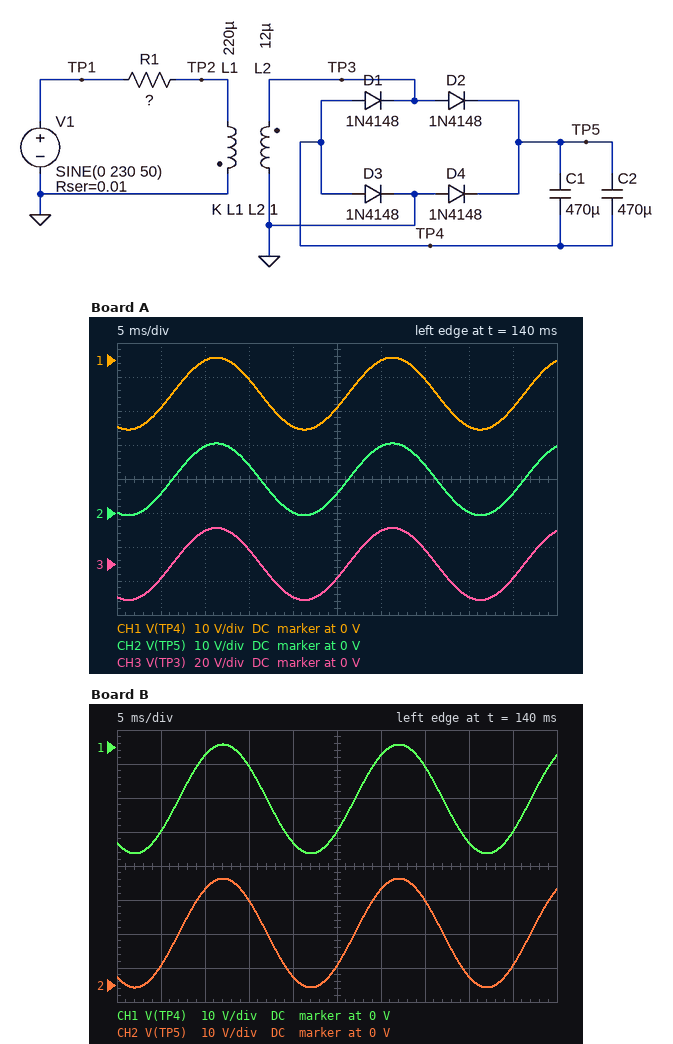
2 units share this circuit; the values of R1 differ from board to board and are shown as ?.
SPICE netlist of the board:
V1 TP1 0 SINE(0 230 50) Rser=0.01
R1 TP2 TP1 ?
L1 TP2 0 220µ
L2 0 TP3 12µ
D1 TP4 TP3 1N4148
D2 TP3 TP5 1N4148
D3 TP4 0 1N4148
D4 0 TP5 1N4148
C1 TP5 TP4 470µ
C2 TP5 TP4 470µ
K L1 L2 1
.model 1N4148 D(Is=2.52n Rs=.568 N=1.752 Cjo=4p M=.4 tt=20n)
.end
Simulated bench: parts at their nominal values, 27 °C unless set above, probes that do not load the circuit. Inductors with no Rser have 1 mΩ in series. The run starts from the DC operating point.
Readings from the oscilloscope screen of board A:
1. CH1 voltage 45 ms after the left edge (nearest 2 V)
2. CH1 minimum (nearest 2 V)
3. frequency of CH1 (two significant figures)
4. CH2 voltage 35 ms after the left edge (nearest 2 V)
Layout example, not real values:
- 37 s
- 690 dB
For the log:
- -14 V
- -20 V
- 50 Hz
- 14 V
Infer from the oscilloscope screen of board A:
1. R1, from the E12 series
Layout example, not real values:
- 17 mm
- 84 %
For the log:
- 0.15 Ω
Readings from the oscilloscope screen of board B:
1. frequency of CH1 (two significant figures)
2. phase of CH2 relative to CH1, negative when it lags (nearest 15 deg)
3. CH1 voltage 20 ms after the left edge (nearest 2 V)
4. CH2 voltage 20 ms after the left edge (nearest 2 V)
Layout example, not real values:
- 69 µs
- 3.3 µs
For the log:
- 50 Hz
- 0 deg
- -28 V
- 2 V
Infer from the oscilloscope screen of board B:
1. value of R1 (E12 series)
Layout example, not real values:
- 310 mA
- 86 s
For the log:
- 0.082 Ω
